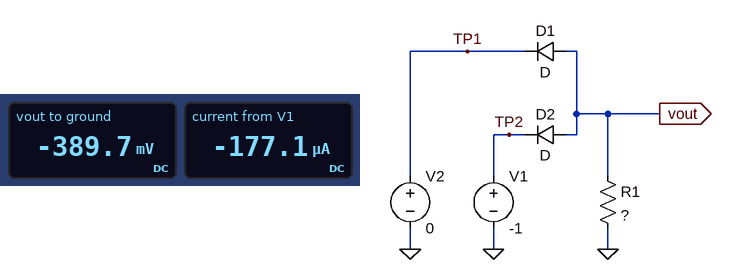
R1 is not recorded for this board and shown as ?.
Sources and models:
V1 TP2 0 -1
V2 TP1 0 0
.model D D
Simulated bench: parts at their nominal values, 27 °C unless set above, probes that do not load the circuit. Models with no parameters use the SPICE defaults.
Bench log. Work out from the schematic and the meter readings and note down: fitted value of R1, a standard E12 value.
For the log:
2.2 kΩ
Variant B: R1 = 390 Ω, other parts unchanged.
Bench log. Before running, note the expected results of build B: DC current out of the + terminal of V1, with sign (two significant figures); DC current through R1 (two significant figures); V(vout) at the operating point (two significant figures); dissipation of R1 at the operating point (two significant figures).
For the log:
-890 µA
890 µA
-350 mV
310 µW
